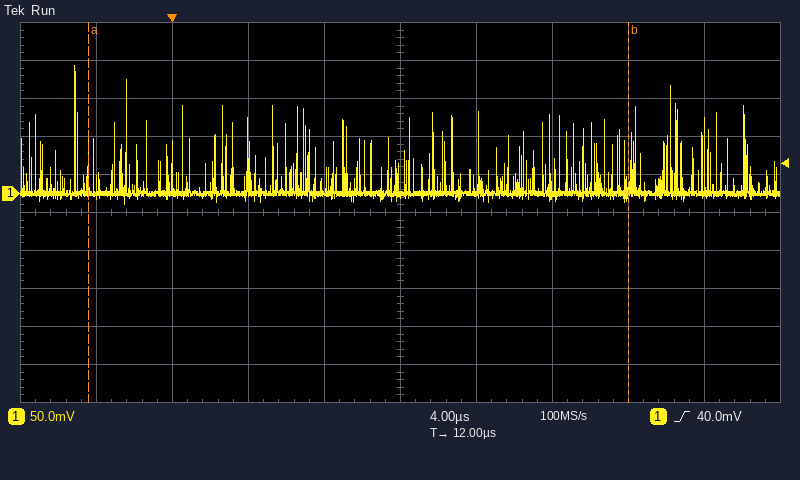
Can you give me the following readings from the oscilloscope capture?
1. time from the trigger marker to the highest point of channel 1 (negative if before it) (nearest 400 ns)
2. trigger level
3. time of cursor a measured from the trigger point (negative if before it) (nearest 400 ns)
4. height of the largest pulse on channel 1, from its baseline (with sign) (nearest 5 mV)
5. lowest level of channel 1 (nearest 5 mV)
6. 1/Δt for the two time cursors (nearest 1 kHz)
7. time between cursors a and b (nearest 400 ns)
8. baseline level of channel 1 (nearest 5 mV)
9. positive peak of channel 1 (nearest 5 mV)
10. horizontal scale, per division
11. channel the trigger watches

-5.2 µs
40.0 mV
-4.4 µs
+170 mV
-15 mV
35 kHz
28.4 µs
0 mV
170 mV
4 µs
channel 1
